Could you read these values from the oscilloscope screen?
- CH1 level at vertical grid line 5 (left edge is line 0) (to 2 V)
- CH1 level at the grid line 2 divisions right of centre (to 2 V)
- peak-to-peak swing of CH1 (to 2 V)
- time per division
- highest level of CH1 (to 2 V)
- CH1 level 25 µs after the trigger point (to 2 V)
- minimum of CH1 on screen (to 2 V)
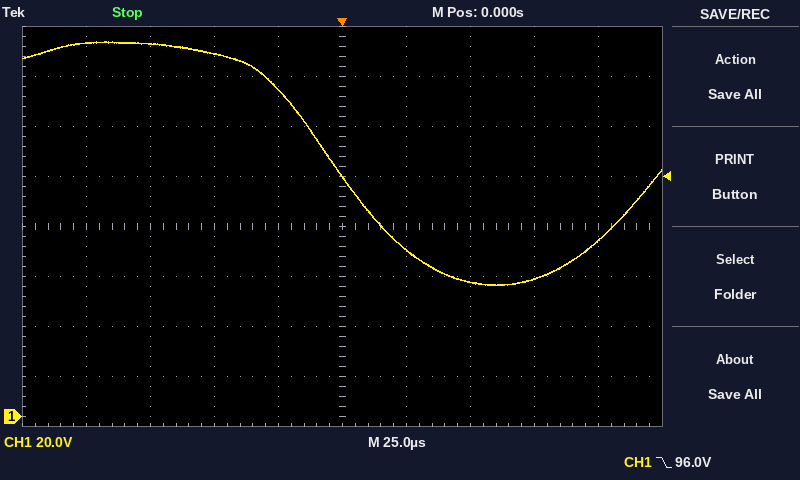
96 V
54 V
98 V
25 µs
150 V
66 V
52 V
